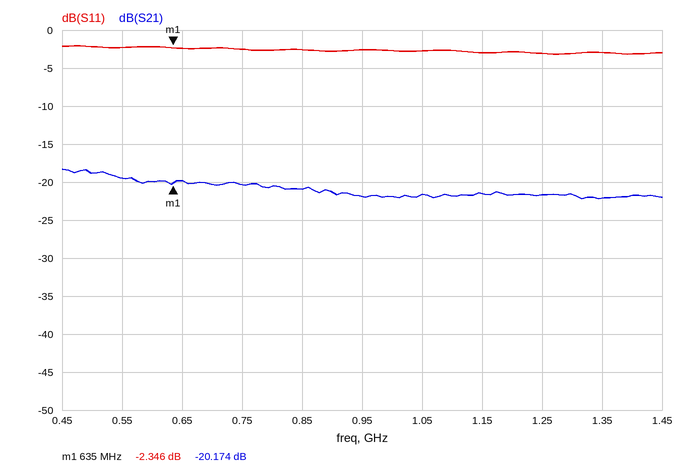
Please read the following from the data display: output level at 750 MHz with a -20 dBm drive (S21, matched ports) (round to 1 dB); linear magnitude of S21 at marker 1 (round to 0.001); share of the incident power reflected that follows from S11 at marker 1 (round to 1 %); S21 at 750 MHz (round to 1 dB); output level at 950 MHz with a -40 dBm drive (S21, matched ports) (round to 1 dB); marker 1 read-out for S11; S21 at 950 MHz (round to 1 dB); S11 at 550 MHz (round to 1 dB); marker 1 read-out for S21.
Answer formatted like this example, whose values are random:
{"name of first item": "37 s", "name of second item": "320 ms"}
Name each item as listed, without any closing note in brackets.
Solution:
{"output level at 750 MHz with a -20 dBm drive (S21, matched ports)": "-40 dBm", "linear magnitude of S21 at marker 1": "0.098", "share of the incident power reflected that follows from S11 at marker 1": "58 %", "S21 at 750 MHz": "-20 dB", "output level at 950 MHz with a -40 dBm drive (S21, matched ports)": "-62 dBm", "marker 1 read-out for S11": "-2.346 dB", "S21 at 950 MHz": "-22 dB", "S11 at 550 MHz": "-2 dB", "marker 1 read-out for S21": "-20.174 dB"}
